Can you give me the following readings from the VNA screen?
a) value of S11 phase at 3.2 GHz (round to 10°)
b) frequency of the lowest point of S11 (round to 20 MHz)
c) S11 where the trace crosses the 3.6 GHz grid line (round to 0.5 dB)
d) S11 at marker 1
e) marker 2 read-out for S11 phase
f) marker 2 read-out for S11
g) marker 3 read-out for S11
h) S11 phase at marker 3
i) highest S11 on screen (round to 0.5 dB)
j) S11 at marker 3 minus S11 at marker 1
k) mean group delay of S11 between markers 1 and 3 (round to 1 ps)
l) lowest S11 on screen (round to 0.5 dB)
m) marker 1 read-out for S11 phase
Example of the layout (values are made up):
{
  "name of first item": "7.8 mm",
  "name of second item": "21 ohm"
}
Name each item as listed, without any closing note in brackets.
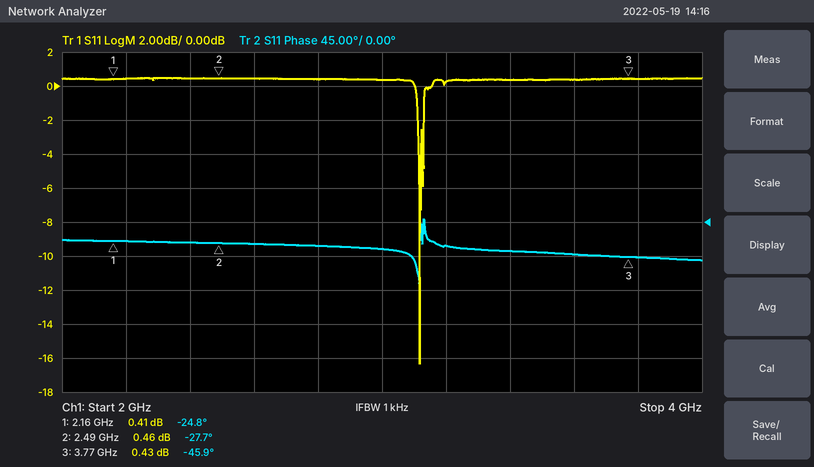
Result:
{
  "value of S11 phase at 3.2 GHz": "-30°",
  "frequency of the lowest point of S11": "3.12 GHz",
  "S11 where the trace crosses the 3.6 GHz grid line": "0.5 dB",
  "S11 at marker 1": "0.41 dB",
  "marker 2 read-out for S11 phase": "-27.7°",
  "marker 2 read-out for S11": "0.46 dB",
  "marker 3 read-out for S11": "0.43 dB",
  "S11 phase at marker 3": "-45.9°",
  "highest S11 on screen": "0.5 dB",
  "S11 at marker 3 minus S11 at marker 1": "0.02 dB",
  "mean group delay of S11 between markers 1 and 3": "36 ps",
  "lowest S11 on screen": "-16.5 dB",
  "marker 1 read-out for S11 phase": "-24.8°"
}
